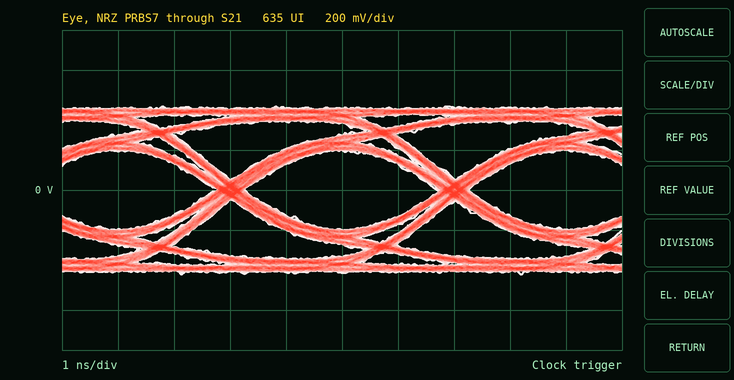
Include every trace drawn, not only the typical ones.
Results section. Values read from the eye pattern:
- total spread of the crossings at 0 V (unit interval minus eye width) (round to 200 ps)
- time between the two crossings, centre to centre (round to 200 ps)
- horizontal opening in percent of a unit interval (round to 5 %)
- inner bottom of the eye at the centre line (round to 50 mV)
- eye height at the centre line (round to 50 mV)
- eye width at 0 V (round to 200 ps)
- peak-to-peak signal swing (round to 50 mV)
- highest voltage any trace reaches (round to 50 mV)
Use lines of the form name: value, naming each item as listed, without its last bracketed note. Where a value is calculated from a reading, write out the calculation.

total spread of the crossings at 0 V (unit interval minus eye width): 600 ps
time between the two crossings, centre to centre: 4.0 ns
horizontal opening in percent of a unit interval: 3.4 ns / 4.0 ns ≈ 85 %
inner bottom of the eye at the centre line: -200 mV
eye height at the centre line: 400 mV
eye width at 0 V: 3.4 ns
peak-to-peak signal swing: 850 mV
highest voltage any trace reaches: 400 mV
